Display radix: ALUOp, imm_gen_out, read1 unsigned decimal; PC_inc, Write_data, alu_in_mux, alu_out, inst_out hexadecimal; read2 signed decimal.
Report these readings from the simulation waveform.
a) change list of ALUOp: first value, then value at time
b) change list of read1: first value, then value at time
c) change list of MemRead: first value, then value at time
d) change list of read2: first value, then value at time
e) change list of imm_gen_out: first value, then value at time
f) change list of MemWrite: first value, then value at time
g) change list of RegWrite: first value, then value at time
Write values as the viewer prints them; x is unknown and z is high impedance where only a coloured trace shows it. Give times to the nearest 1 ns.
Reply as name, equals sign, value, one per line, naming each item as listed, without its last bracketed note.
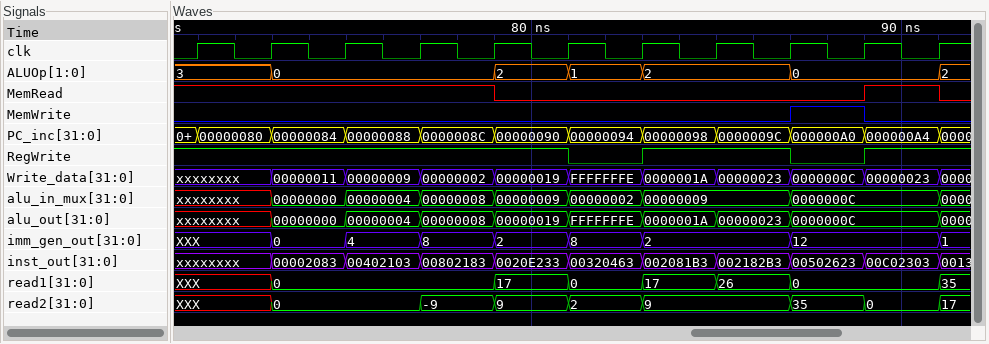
change list of ALUOp: first value, then value at time = 3, 0 at 73 ns, 2 at 79 ns, 1 at 81 ns, 2 at 83 ns, 0 at 87 ns, 2 at 91 ns
change list of read1: first value, then value at time = XXX, 0 at 73 ns, 17 at 79 ns, 0 at 81 ns, 17 at 83 ns, 26 at 85 ns, 0 at 87 ns, 35 at 91 ns
change list of MemRead: first value, then value at time = 1, 0 at 79 ns, 1 at 89 ns, 0 at 91 ns
change list of read2: first value, then value at time = XXX, 0 at 73 ns, -9 at 77 ns, 9 at 79 ns, 2 at 81 ns, 9 at 83 ns, 35 at 87 ns, 0 at 89 ns, 17 at 91 ns
change list of imm_gen_out: first value, then value at time = XXX, 0 at 73 ns, 4 at 75 ns, 8 at 77 ns, 2 at 79 ns, 8 at 81 ns, 2 at 83 ns, 12 at 87 ns, 1 at 91 ns
change list of MemWrite: first value, then value at time = 0, 1 at 87 ns, 0 at 89 ns
change list of RegWrite: first value, then value at time = 1, 0 at 81 ns, 1 at 83 ns, 0 at 87 ns, 1 at 89 ns
